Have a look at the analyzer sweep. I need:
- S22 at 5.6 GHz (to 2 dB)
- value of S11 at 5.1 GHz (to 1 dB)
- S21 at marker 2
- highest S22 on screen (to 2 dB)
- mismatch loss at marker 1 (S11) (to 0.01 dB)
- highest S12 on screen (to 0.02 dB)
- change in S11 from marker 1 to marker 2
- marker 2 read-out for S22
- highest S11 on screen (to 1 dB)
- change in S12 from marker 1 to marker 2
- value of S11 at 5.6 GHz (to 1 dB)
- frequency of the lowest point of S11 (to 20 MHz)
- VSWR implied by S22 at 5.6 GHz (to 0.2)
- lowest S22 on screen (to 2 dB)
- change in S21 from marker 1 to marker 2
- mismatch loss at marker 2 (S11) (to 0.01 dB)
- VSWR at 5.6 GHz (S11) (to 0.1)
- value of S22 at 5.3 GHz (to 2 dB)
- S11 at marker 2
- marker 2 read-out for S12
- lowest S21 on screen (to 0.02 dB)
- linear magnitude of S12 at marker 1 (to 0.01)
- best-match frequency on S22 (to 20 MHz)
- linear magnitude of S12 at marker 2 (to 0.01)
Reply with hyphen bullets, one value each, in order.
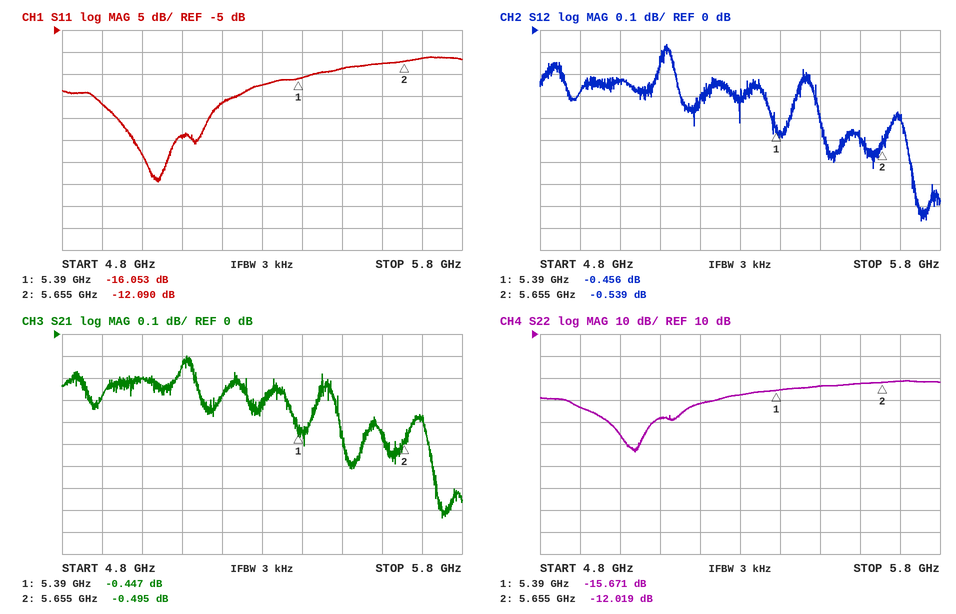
- -12 dB
- -29 dB
- -0.495 dB
- -12 dB
- 0.11 dB
- -0.06 dB
- 3.963 dB
- -12.019 dB
- -11 dB
- -0.083 dB
- -13 dB
- 5.04 GHz
- 1.6
- -44 dB
- -0.048 dB
- 0.28 dB
- 1.6
- -18 dB
- -12.090 dB
- -0.539 dB
- -0.84 dB
- 0.95
- 5.04 GHz
- 0.94
